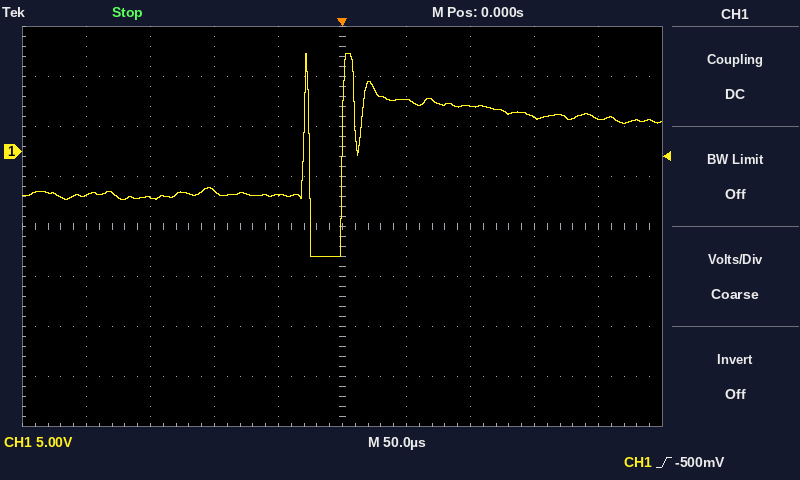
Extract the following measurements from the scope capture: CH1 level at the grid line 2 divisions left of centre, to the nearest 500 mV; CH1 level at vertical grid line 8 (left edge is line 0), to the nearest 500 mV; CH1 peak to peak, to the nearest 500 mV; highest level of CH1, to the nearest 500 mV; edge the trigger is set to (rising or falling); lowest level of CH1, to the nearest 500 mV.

-4.0 V
3.5 V
20.5 V
10.0 V
rising
-10.5 V
